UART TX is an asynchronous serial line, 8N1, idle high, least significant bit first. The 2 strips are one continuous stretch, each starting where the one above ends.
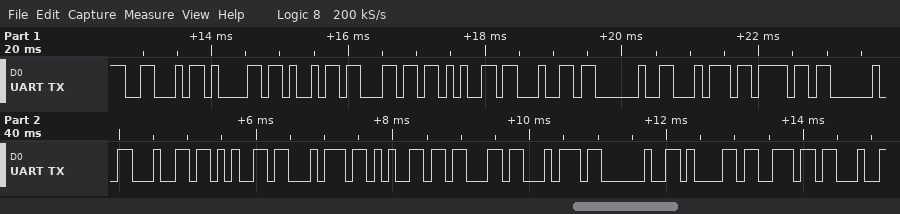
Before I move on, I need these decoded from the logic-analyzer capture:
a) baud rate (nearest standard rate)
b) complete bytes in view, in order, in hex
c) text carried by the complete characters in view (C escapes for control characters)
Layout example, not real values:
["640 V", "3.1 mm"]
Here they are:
["9600 baud", "46 61 69 6C 65 64 20 74 6F 20 64 65 74 65 63 74 20 61 6E", "\"Failed to detect an\""]
